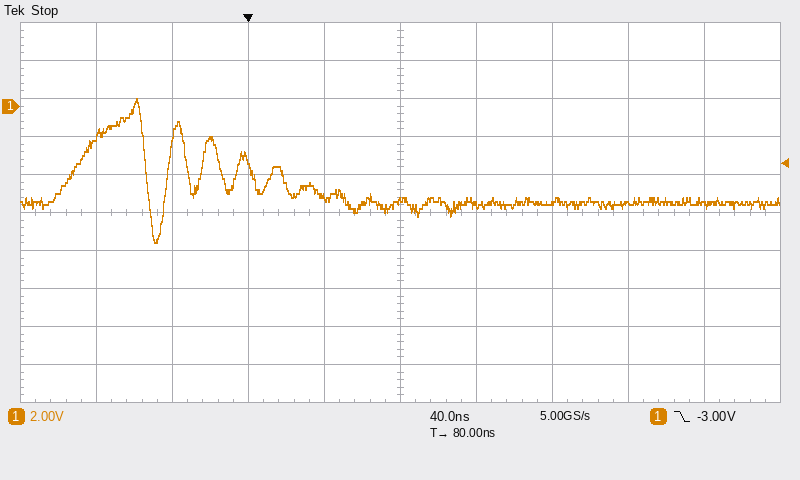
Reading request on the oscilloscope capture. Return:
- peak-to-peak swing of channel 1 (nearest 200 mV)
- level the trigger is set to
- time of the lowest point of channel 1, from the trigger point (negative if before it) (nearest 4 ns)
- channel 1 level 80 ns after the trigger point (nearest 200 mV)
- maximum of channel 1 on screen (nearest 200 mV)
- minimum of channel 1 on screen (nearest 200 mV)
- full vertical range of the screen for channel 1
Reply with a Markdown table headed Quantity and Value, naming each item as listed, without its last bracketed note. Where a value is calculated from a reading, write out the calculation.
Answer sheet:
| Quantity | Value |
|---|---|
| peak-to-peak swing of channel 1 | 400 mV − (-7.2 V) = 7.6 V |
| level the trigger is set to | -3.00 V |
| time of the lowest point of channel 1, from the trigger point (negative if before it) | -48 ns |
| channel 1 level 80 ns after the trigger point | -5.0 V |
| maximum of channel 1 on screen | 400 mV |
| minimum of channel 1 on screen | -7.2 V |
| full vertical range of the screen for channel 1 | 20 V |
